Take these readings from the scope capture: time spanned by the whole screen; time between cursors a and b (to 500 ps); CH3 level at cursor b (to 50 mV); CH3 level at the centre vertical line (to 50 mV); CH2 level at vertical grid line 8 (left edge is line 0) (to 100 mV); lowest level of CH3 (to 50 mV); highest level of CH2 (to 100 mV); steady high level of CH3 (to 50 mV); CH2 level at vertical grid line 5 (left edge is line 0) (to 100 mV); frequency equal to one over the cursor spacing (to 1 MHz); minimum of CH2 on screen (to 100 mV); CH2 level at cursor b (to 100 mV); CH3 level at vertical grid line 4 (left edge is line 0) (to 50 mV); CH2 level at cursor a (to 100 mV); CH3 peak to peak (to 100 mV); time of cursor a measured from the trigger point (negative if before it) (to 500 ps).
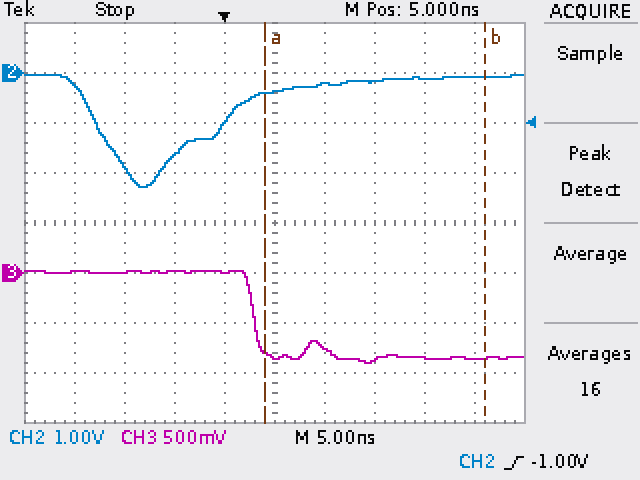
50 ns
22.0 ns
-850 mV
-850 mV
-100 mV
-900 mV
0.0 V
0 mV
-400 mV
45 MHz
-2.3 V
-100 mV
0 mV
-400 mV
900 mV
+4.0 ns
